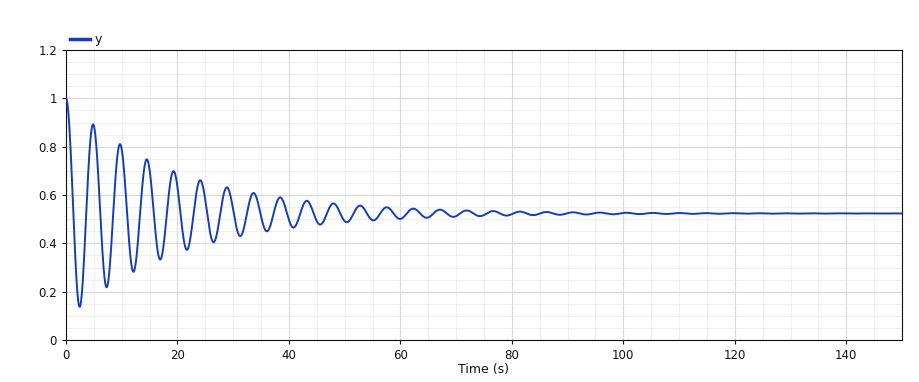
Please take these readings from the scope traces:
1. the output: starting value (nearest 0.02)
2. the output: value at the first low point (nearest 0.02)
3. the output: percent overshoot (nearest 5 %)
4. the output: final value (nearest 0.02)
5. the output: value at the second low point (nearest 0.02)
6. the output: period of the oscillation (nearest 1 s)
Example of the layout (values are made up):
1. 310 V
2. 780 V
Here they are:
1. 1.00
2. 0.14
3. 80 %
4. 0.52
5. 0.22
6. 5 s
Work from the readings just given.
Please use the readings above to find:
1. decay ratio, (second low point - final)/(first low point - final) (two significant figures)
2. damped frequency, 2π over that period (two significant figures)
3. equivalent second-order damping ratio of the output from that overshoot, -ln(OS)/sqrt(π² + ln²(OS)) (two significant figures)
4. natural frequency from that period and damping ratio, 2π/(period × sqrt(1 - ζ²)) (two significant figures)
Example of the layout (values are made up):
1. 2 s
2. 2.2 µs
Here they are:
1. 0.79
2. 1.3 rad/s
3. 0.071
4. 1.3 rad/s
